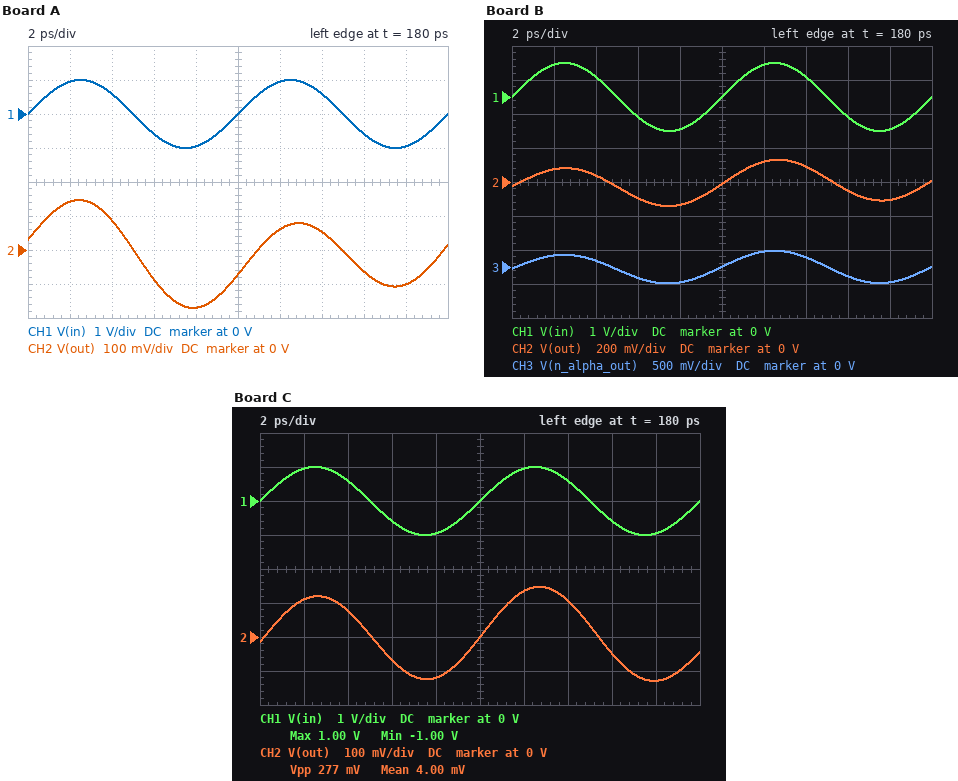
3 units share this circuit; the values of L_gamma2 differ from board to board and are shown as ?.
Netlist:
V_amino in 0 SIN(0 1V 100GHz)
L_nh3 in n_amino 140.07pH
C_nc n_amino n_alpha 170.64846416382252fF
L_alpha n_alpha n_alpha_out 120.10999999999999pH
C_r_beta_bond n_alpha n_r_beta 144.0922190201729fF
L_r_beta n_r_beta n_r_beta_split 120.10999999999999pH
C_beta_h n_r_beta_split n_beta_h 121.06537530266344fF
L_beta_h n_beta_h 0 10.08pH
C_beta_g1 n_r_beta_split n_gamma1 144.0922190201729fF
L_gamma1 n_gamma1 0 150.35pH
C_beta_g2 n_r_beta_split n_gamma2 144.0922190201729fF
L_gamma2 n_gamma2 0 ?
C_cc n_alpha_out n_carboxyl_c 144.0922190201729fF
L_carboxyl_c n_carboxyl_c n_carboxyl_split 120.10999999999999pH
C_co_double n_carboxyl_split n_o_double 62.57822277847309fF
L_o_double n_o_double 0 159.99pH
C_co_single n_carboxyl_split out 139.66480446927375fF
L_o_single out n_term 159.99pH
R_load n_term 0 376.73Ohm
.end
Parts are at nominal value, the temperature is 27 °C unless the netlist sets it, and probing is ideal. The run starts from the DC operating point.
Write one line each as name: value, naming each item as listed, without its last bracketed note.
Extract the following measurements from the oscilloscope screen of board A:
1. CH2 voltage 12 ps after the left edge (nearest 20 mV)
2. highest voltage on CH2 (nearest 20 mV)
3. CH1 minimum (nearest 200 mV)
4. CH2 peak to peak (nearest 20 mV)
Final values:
CH2 voltage 12 ps after the left edge: 60 mV
highest voltage on CH2: 140 mV
CH1 minimum: -1.0 V
CH2 peak to peak: 320 mV
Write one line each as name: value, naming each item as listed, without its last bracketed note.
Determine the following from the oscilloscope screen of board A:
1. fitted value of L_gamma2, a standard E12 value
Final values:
fitted value of L_gamma2, a standard E12 value: 120 pH
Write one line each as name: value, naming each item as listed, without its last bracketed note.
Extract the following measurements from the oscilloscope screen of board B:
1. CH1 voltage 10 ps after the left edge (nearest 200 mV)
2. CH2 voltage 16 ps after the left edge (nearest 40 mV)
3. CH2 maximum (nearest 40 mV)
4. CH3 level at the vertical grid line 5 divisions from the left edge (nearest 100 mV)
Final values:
CH1 voltage 10 ps after the left edge: 0 V
CH2 voltage 16 ps after the left edge: -40 mV
CH2 maximum: 120 mV
CH3 level at the vertical grid line 5 divisions from the left edge: 0 V
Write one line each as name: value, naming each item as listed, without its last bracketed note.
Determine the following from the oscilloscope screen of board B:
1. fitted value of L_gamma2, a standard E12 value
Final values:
fitted value of L_gamma2, a standard E12 value: 100 pH
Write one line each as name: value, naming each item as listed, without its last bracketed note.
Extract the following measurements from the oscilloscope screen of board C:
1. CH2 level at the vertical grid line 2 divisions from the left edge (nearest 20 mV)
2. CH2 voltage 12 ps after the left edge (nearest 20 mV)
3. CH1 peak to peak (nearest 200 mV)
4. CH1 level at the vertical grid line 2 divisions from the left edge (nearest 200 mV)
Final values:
CH2 level at the vertical grid line 2 divisions from the left edge: 80 mV
CH2 voltage 12 ps after the left edge: 140 mV
CH1 peak to peak: 2.0 V
CH1 level at the vertical grid line 2 divisions from the left edge: 600 mV
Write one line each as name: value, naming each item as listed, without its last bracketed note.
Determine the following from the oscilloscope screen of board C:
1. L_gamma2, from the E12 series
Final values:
L_gamma2, from the E12 series: 82 pH
